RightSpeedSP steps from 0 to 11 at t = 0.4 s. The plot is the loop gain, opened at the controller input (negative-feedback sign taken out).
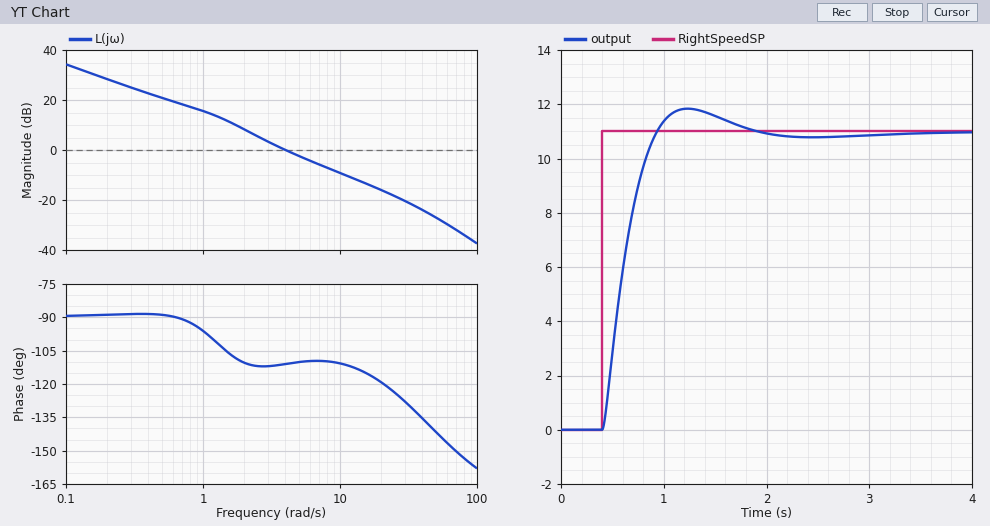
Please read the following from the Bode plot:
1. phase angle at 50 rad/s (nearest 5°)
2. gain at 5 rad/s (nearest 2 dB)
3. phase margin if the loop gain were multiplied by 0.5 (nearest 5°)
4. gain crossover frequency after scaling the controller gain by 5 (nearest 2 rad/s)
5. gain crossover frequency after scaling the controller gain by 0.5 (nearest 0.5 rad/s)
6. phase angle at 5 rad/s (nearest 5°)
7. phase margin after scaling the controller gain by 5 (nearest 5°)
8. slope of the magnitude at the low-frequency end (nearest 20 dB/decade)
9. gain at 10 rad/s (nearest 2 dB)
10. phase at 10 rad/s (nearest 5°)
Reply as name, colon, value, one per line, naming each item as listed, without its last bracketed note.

phase angle at 50 rad/s: -140°
gain at 5 rad/s: -2 dB
phase margin if the loop gain were multiplied by 0.5: 70°
gain crossover frequency after scaling the controller gain by 5: 16 rad/s
gain crossover frequency after scaling the controller gain by 0.5: 2.5 rad/s
phase angle at 5 rad/s: -110°
phase margin after scaling the controller gain by 5: 65°
slope of the magnitude at the low-frequency end: -20 dB/decade
gain at 10 rad/s: -10 dB
phase at 10 rad/s: -110°
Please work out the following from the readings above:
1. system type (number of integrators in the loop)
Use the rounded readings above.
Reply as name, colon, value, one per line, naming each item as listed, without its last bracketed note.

system type: 1
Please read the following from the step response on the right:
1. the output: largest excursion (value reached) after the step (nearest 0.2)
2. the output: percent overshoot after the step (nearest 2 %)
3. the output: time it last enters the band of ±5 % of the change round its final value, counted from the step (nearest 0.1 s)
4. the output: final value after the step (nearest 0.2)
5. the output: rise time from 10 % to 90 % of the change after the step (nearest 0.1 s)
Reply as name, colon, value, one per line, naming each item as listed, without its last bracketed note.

the output: largest excursion (value reached) after the step: 11.8
the output: percent overshoot after the step: 8 %
the output: time it last enters the band of ±5 % of the change round its final value, counted from the step: 1.1 s
the output: final value after the step: 11.0
the output: rise time from 10 % to 90 % of the change after the step: 0.4 s
